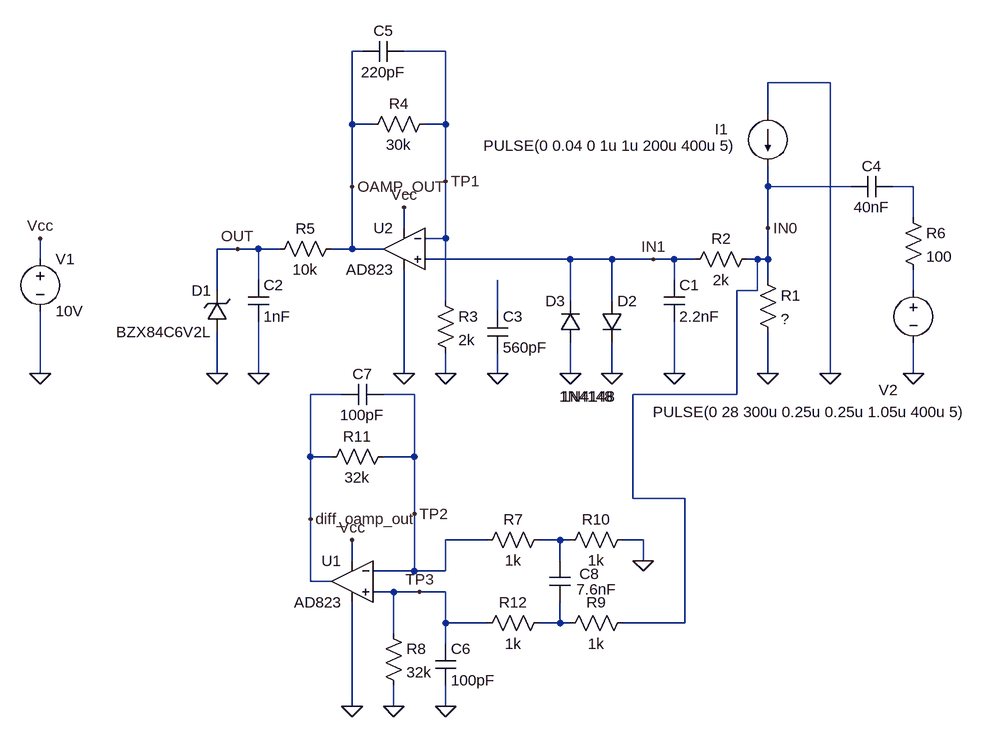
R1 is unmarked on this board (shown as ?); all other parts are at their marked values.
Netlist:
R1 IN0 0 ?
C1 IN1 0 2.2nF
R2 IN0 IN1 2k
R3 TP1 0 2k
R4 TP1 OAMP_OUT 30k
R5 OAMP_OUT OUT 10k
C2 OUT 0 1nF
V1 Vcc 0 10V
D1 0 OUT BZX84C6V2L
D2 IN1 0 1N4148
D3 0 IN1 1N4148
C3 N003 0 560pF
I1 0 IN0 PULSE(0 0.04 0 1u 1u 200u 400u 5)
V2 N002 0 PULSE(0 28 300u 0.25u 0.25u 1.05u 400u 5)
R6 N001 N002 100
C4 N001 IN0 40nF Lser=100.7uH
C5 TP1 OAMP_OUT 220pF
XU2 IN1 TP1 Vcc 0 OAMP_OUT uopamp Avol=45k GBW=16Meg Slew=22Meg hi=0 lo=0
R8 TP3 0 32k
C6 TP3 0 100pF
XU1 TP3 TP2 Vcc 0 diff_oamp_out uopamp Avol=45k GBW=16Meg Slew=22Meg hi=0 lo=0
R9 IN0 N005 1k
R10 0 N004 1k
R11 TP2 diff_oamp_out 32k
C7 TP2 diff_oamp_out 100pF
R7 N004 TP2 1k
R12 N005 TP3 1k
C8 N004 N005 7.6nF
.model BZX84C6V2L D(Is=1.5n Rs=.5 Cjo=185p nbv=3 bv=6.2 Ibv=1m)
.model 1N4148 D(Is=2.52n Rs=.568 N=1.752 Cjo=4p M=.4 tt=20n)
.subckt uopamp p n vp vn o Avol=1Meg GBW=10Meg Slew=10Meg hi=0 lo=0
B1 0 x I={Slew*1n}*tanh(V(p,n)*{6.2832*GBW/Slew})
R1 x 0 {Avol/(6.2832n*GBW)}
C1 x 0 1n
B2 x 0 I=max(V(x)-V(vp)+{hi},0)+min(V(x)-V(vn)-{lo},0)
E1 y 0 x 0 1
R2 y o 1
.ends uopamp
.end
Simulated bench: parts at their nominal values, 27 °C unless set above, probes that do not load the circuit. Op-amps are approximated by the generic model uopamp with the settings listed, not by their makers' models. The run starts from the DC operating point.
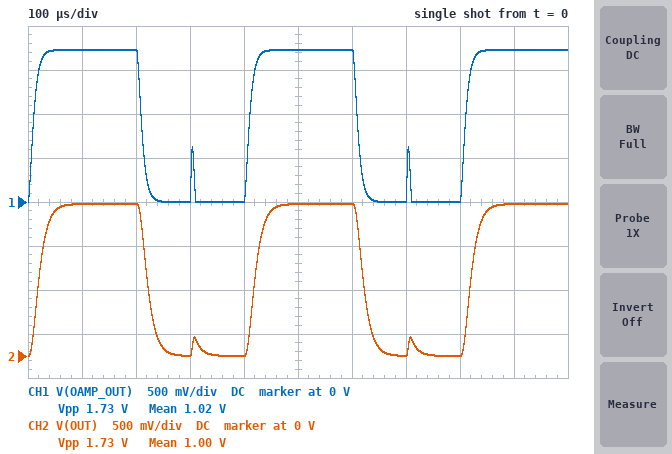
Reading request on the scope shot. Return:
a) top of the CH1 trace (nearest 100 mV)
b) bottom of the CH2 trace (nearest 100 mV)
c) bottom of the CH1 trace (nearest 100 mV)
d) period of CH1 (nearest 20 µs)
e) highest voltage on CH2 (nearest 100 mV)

1.7 V
0 V
0 V
400 µs
1.7 V
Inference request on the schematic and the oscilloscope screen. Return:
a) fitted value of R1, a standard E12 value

2.7 Ω
